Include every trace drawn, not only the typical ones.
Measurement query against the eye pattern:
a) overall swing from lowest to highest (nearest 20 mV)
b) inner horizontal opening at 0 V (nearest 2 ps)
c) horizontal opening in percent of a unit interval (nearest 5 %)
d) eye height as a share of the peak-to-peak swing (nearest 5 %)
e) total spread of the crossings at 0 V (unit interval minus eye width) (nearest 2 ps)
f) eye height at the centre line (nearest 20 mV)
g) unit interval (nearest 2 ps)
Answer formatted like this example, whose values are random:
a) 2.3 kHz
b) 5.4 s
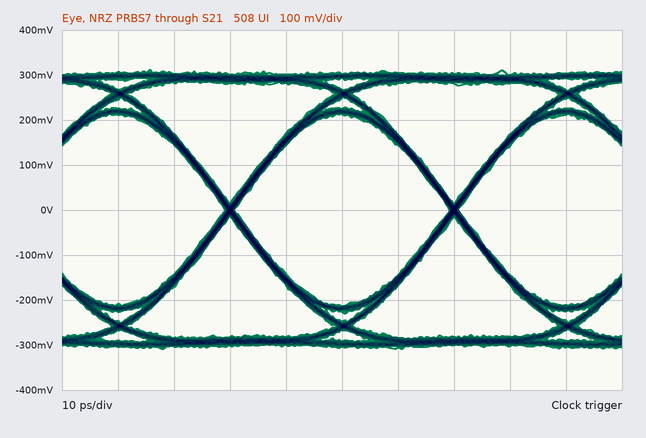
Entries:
a) 620 mV
b) 38 ps
c) 95 %
d) 70 %
e) 2 ps
f) 420 mV
g) 40 ps
